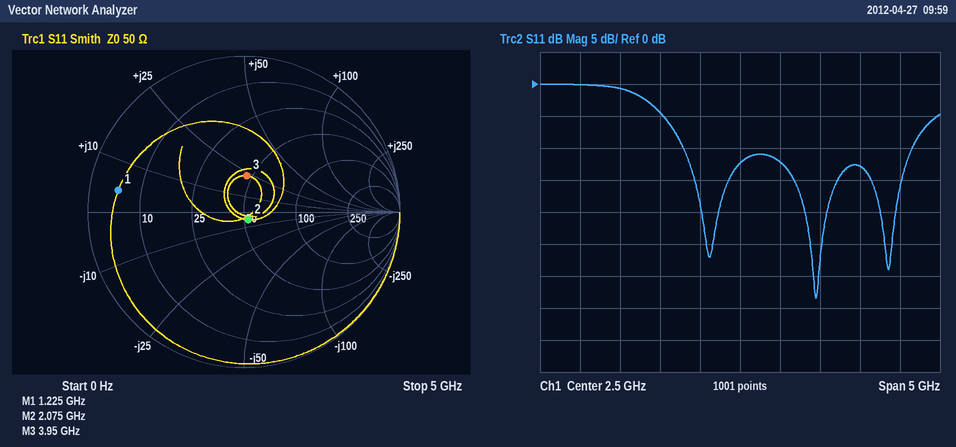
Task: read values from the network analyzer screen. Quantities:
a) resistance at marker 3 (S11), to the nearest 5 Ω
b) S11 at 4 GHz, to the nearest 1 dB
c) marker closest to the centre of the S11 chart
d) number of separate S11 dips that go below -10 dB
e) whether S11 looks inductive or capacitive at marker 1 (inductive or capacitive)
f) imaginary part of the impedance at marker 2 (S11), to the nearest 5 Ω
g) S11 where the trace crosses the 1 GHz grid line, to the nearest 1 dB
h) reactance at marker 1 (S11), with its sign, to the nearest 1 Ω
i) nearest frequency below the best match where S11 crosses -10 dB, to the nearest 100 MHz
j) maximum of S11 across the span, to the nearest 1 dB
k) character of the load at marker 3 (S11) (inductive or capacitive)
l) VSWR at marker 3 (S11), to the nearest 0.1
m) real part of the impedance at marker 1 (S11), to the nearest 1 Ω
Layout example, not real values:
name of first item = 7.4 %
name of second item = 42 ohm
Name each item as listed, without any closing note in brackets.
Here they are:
resistance at marker 3 (S11), to the nearest 5 Ω = 45 Ω
S11 at 4 GHz, to the nearest 1 dB = -13 dB
marker closest to the centre of the S11 chart = marker 2
number of separate S11 dips that go below -10 dB = 3
whether S11 looks inductive or capacitive at marker 1 = inductive
imaginary part of the impedance at marker 2 (S11), to the nearest 5 Ω = -5 Ω
S11 where the trace crosses the 1 GHz grid line, to the nearest 1 dB = -1 dB
reactance at marker 1 (S11), with its sign, to the nearest 1 Ω = +4 Ω
nearest frequency below the best match where S11 crosses -10 dB, to the nearest 100 MHz = 1.8 GHz
maximum of S11 across the span, to the nearest 1 dB = 0 dB
character of the load at marker 3 (S11) = inductive
VSWR at marker 3 (S11), to the nearest 0.1 = 1.6
real part of the impedance at marker 1 (S11), to the nearest 1 Ω = 5 Ω
